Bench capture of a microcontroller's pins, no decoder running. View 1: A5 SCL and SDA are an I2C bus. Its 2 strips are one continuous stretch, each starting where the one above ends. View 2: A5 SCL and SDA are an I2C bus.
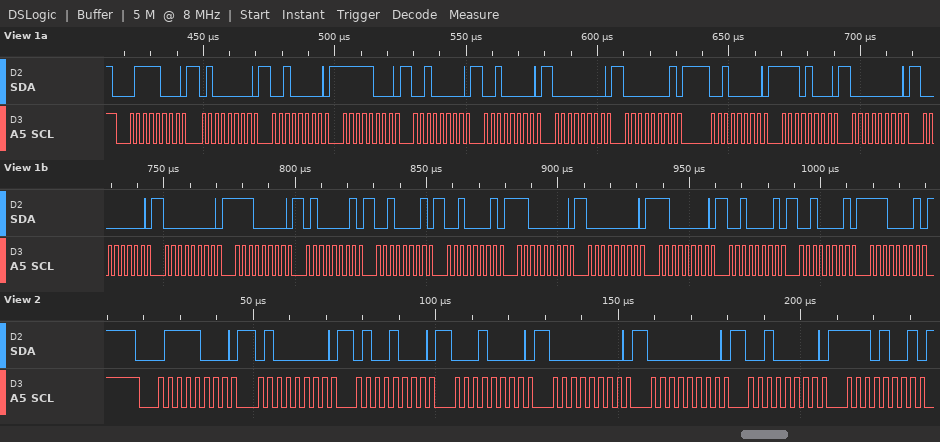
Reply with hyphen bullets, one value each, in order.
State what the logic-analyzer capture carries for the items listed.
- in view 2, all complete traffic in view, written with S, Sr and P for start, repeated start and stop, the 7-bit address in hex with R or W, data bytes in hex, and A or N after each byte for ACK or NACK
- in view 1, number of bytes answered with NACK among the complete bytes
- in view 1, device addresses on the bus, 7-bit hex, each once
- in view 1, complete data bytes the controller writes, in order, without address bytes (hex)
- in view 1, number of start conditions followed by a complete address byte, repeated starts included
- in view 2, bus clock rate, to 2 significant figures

- S 3CW A 40 A 48 A 10 A 00 A 00 A 20 A E9 A
- 0
- 0x3C
- 40 20 F8 20 20 00 01 20 E8 00 00 00 E0 41 21 21 C0 00 C0 21 21 E1
- 1
- 400 kHz
